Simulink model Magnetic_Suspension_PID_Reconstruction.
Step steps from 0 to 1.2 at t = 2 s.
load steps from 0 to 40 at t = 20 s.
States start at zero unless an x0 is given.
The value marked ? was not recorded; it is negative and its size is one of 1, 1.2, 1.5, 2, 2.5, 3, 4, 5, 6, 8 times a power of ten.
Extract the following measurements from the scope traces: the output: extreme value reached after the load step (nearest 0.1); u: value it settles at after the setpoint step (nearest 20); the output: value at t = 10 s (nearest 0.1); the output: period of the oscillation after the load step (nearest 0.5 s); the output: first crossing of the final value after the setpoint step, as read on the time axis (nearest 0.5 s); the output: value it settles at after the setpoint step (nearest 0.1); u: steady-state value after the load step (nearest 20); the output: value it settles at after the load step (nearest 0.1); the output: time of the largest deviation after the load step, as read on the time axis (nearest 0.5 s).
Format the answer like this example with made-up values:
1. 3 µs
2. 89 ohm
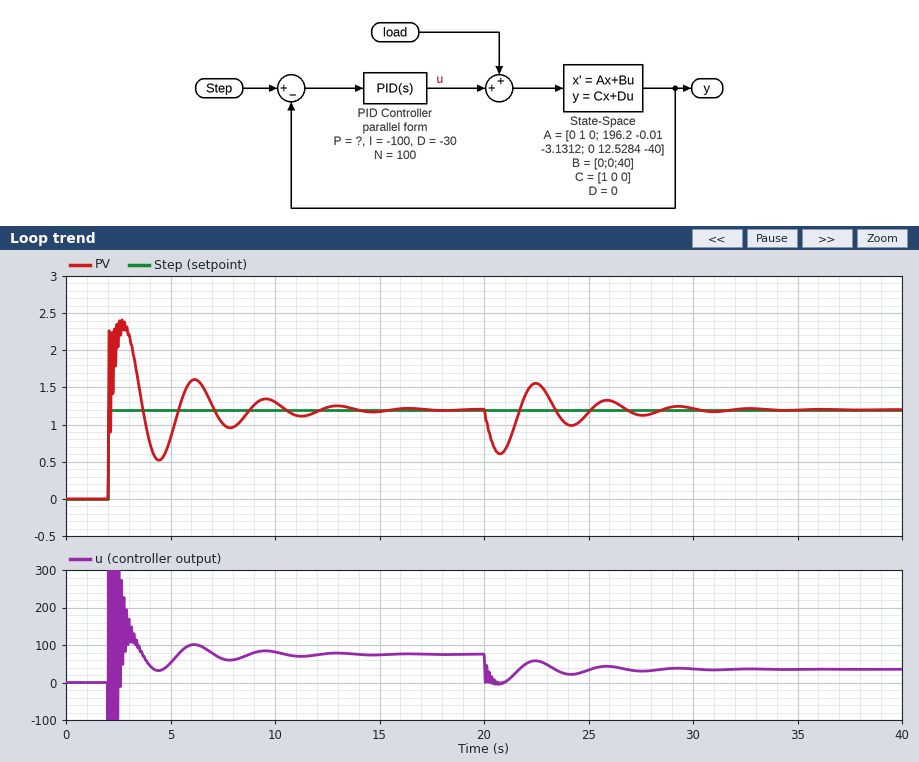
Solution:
1. 0.6
2. 80
3. 1.3
4. 3.5 s
5. 2.0 s
6. 1.2
7. 40
8. 1.2
9. 21.0 s
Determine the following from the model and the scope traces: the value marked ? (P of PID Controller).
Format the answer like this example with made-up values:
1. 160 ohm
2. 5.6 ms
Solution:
1. -80
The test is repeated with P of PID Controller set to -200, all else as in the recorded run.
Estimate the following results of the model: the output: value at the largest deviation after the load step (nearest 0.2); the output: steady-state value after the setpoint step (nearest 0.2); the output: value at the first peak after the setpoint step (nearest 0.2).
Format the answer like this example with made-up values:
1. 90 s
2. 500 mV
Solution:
1. 1.0
2. 1.2
3. 2.4
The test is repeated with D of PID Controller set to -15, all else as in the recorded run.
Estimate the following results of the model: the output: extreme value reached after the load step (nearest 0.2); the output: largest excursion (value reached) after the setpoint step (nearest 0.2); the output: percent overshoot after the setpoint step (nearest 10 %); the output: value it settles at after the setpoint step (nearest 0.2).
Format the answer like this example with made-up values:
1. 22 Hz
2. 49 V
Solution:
1. 0.4
2. 2.8
3. 130 %
4. 1.2
